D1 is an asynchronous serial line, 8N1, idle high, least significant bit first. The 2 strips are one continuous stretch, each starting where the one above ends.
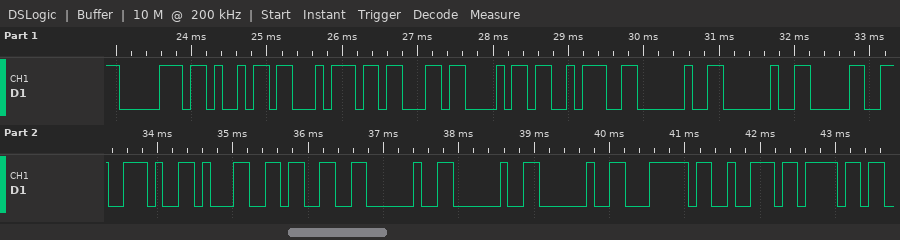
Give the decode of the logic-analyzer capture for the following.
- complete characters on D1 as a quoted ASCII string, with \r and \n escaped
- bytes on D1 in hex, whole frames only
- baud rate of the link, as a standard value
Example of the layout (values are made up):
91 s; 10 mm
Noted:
"pitch:  0.13   |ro"; 70 69 74 63 68 3A 20 20 30 2E 31 33 20 20 20 7C 72 6F; 9600 baud
